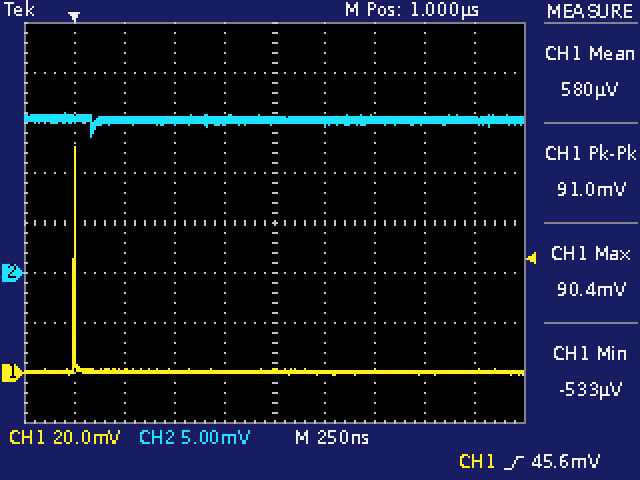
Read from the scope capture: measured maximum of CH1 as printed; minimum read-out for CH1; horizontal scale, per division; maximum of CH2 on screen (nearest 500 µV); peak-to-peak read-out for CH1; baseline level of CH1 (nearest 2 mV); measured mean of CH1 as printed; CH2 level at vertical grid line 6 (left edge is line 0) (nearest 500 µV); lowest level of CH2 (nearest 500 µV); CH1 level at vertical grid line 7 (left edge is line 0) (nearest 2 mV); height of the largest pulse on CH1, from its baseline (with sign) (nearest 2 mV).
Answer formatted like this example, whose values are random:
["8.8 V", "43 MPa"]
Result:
["90.4 mV", "-533 µV", "250 ns", "16.0 mV", "91.0 mV", "0 mV", "580 µV", "15.0 mV", "13.5 mV", "0 mV", "+90 mV"]
